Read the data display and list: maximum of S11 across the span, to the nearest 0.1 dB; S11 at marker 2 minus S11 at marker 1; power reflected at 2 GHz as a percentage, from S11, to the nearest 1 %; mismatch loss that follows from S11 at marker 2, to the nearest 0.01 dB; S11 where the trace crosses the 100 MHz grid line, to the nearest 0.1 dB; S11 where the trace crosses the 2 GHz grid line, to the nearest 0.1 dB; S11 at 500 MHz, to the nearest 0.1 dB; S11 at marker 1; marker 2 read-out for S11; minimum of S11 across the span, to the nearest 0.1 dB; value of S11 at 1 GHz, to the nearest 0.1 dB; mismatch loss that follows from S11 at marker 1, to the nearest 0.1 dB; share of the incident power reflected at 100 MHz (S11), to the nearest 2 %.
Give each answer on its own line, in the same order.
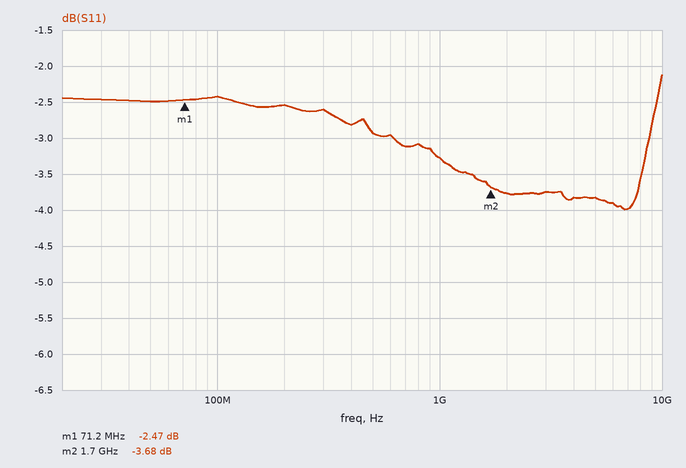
-2.1 dB
-1.21 dB
42 %
2.43 dB
-2.4 dB
-3.8 dB
-2.9 dB
-2.47 dB
-3.68 dB
-4.0 dB
-3.3 dB
3.6 dB
58 %
